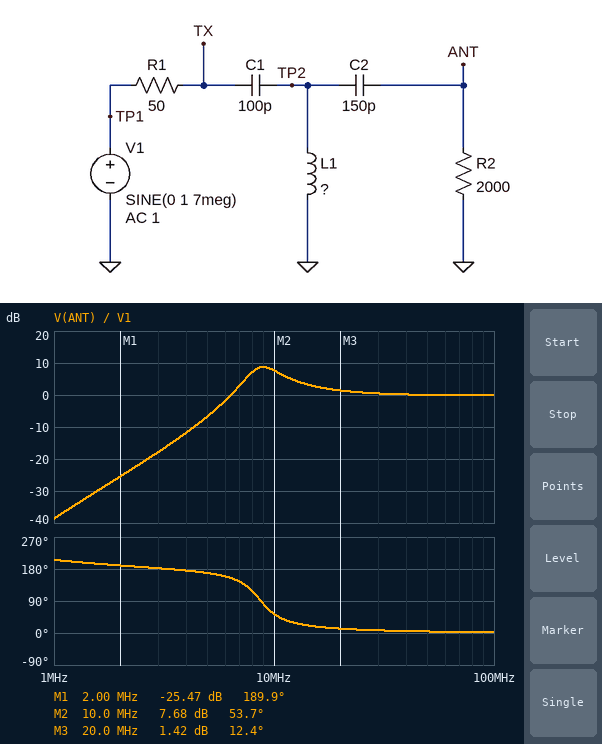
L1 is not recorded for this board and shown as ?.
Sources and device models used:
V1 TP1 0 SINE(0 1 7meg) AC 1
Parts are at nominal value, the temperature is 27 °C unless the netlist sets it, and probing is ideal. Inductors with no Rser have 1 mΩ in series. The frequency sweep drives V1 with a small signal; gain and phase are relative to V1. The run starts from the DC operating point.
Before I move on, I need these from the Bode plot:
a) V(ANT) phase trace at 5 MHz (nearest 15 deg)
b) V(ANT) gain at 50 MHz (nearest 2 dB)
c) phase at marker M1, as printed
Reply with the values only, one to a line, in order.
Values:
165 deg
0 dB
189.9 deg
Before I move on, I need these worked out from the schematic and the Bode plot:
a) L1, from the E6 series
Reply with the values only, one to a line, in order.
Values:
3.3 µH
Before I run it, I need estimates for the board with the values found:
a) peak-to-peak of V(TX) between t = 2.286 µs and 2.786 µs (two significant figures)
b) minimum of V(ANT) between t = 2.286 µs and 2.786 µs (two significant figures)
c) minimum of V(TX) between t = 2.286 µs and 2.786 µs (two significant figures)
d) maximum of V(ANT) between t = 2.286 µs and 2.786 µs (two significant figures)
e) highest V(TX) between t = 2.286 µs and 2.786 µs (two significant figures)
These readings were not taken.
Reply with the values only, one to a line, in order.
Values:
1.6 V
-1.4 V
-810 mV
1.4 V
810 mV
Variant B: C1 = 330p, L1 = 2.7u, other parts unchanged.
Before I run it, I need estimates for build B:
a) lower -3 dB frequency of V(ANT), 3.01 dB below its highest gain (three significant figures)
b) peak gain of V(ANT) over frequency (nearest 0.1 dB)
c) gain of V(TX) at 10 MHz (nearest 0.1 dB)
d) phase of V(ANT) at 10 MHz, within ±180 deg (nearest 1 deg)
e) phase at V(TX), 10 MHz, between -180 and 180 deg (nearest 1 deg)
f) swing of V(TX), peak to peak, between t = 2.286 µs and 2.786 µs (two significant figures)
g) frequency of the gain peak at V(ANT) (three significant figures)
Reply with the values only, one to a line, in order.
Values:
4.46 MHz
4.7 dB
-1.0 dB
26 deg
21 deg
1.3 V
5.79 MHz
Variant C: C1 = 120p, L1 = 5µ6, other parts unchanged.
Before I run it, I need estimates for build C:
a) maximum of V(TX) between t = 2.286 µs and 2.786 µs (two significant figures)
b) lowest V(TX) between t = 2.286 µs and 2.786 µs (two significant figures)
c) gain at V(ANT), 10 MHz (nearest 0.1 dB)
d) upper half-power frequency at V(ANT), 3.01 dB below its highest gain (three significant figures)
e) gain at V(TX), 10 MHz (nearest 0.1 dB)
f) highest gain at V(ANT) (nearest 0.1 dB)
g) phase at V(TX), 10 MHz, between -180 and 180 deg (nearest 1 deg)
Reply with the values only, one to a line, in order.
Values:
650 mV
-650 mV
3.3 dB
7.70 MHz
-0.7 dB
9.4 dB
12 deg
